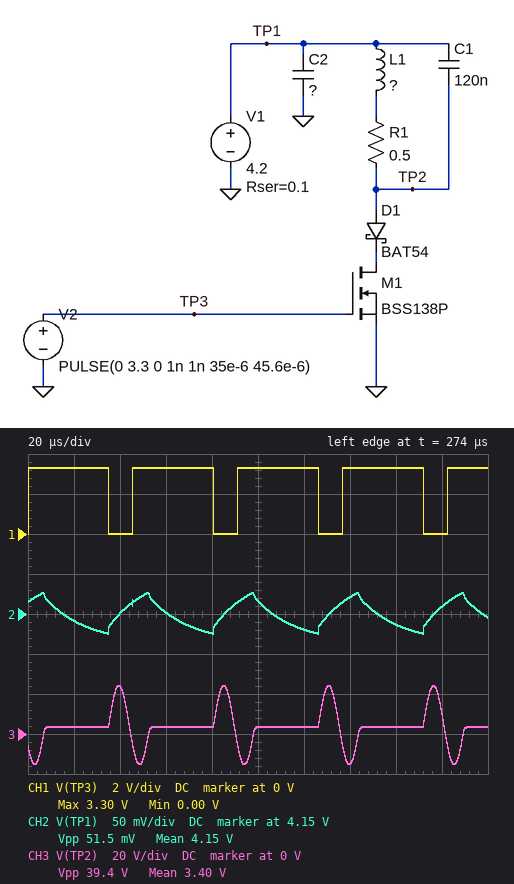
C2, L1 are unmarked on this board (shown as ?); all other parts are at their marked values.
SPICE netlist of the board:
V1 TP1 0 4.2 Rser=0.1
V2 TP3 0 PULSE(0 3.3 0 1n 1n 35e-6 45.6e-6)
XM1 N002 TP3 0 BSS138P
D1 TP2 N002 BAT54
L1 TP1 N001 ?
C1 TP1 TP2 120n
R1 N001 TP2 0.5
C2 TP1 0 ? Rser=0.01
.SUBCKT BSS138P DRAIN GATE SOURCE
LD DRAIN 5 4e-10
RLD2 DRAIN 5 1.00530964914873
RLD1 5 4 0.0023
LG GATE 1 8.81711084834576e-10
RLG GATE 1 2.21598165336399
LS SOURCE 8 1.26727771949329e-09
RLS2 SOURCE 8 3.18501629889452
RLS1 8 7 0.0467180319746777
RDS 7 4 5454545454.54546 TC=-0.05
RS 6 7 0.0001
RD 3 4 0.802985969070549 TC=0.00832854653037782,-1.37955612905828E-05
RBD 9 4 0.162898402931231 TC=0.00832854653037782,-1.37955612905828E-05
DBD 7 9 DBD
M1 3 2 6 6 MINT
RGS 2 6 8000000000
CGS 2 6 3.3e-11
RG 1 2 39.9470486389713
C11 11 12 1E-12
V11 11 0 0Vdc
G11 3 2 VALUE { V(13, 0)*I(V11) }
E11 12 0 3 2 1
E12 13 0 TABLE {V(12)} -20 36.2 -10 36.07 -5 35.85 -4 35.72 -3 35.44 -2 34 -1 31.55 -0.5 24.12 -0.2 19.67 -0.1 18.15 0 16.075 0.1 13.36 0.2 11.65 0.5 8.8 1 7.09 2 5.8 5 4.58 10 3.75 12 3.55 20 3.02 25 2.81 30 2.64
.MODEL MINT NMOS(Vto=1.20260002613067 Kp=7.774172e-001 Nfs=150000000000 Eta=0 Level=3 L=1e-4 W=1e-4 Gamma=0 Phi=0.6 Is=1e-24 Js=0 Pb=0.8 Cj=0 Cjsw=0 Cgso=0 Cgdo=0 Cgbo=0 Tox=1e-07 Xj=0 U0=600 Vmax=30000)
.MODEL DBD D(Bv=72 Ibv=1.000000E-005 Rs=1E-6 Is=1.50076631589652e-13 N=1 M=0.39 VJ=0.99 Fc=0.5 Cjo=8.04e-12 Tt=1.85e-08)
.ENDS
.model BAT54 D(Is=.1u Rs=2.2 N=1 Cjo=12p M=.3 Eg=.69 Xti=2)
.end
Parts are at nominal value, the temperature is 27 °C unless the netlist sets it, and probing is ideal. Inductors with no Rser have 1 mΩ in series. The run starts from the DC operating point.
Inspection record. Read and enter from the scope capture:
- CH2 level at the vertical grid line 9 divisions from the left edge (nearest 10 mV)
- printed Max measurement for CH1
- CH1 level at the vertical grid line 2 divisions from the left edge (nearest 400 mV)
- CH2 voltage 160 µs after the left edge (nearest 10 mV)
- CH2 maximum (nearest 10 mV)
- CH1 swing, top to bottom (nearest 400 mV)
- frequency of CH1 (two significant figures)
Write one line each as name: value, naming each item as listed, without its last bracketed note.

CH2 level at the vertical grid line 9 divisions from the left edge: 4.16 V
printed Max measurement for CH1: 3.30 V
CH1 level at the vertical grid line 2 divisions from the left edge: 0 V
CH2 voltage 160 µs after the left edge: 4.14 V
CH2 maximum: 4.18 V
CH1 swing, top to bottom: 3.2 V
frequency of CH1: 22 kHz
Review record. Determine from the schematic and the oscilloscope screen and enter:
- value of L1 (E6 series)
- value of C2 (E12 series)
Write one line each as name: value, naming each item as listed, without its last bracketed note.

value of L1: 68 µH
value of C2: 150 µF
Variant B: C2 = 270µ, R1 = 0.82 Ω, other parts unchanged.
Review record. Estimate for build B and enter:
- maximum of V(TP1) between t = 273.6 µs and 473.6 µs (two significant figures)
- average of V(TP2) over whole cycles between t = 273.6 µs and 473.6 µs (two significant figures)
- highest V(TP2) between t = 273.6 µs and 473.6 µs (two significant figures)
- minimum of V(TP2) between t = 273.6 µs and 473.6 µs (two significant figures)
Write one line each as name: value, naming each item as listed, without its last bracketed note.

maximum of V(TP1) between t = 273.6 µs and 473.6 µs: 4.2 V
average of V(TP2) over whole cycles between t = 273.6 µs and 473.6 µs: 3.8 V
highest V(TP2) between t = 273.6 µs and 473.6 µs: 23 V
minimum of V(TP2) between t = 273.6 µs and 473.6 µs: -13 V
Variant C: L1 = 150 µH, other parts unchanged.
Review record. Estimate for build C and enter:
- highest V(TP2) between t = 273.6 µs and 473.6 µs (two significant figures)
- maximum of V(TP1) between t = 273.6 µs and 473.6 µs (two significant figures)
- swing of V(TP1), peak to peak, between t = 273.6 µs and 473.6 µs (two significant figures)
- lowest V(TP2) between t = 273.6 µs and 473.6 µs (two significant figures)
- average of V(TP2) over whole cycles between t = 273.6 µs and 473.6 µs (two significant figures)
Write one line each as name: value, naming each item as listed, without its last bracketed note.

highest V(TP2) between t = 273.6 µs and 473.6 µs: 30 V
maximum of V(TP1) between t = 273.6 µs and 473.6 µs: 4.2 V
swing of V(TP1), peak to peak, between t = 273.6 µs and 473.6 µs: 40 mV
lowest V(TP2) between t = 273.6 µs and 473.6 µs: -17 V
average of V(TP2) over whole cycles between t = 273.6 µs and 473.6 µs: 4.0 V
